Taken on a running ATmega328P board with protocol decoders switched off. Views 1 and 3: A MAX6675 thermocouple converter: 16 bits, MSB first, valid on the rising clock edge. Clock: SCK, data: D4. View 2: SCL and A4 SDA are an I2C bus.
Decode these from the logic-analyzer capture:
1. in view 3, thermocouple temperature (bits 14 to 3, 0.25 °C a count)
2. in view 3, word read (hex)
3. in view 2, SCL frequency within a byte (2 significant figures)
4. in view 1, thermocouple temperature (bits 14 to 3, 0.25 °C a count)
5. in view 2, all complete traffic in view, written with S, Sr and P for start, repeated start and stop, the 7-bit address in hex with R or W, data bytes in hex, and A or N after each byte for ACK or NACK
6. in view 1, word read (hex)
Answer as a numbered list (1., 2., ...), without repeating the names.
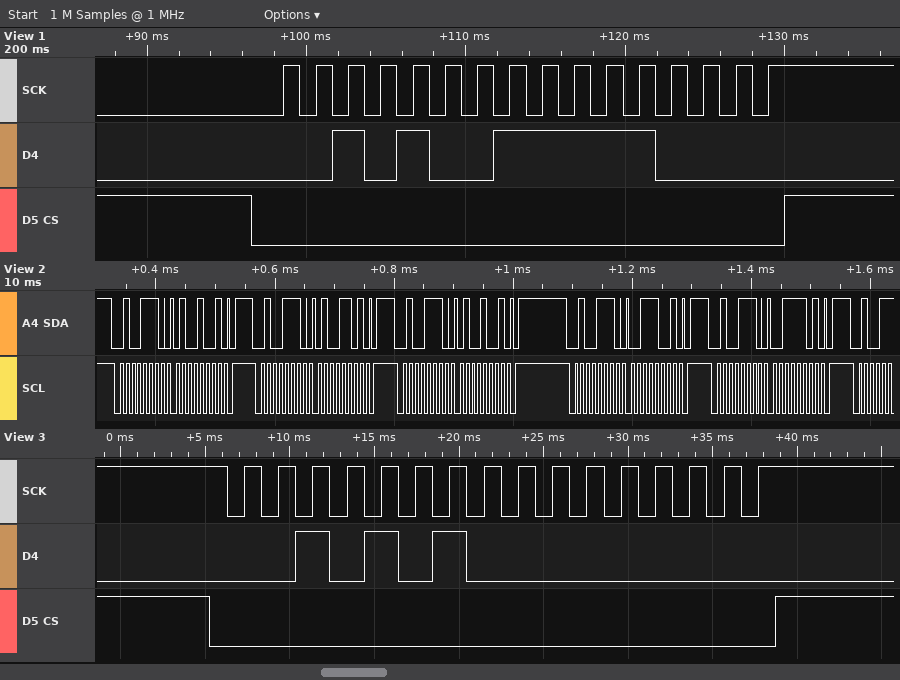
1. 336.00 °C
2. 0x2A00
3. 100 kHz
4. 335.50 °C
5. S 27W A 49 A P S 27W A 4D A P S 27W A 49 A P S 27W A 39 A P S 27W A 3D A P
6. 0x29F0
